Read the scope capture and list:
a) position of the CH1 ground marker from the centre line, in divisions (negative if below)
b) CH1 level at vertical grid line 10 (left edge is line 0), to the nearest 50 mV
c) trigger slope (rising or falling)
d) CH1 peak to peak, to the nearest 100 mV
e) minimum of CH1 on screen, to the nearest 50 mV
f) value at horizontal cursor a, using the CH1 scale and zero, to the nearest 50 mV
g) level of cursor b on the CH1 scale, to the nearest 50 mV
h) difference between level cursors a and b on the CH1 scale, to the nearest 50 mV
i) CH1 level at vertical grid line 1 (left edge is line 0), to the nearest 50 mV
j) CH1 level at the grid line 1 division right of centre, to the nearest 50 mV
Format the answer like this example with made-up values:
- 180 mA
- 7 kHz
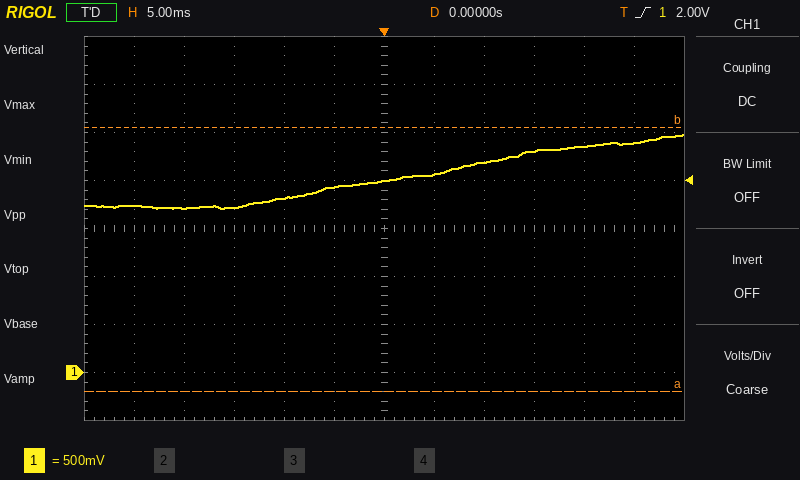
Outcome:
- -3.0 div
- 2.35 V
- rising
- 800 mV
- 1.70 V
- -200 mV
- 2.55 V
- 2.75 V
- 1.75 V
- 2.05 V
